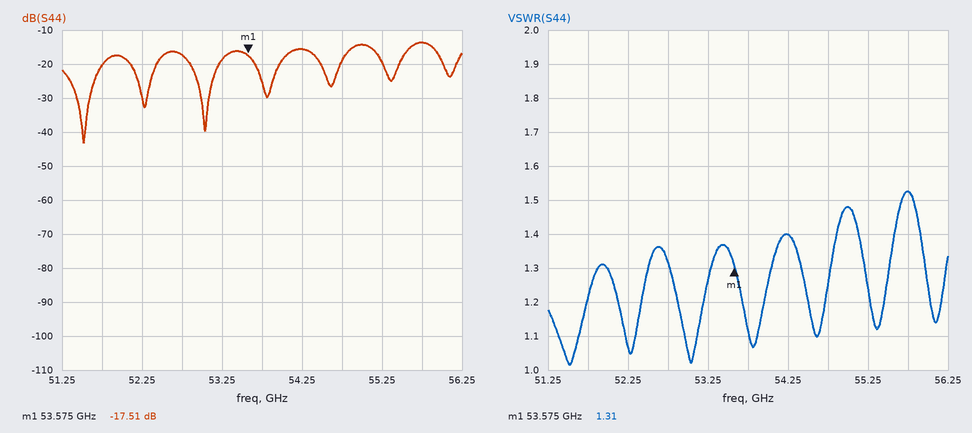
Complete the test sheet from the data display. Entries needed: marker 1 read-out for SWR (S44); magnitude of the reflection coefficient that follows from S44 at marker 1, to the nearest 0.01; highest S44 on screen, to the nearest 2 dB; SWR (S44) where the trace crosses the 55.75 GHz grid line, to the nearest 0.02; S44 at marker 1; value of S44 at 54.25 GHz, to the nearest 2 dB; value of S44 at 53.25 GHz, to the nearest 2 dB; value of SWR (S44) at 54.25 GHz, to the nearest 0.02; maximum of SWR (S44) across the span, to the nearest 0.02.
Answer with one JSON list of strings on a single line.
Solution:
["1.31", "0.13", "-14 dB", "1.52", "-17.51 dB", "-16 dB", "-18 dB", "1.40", "1.52"]
